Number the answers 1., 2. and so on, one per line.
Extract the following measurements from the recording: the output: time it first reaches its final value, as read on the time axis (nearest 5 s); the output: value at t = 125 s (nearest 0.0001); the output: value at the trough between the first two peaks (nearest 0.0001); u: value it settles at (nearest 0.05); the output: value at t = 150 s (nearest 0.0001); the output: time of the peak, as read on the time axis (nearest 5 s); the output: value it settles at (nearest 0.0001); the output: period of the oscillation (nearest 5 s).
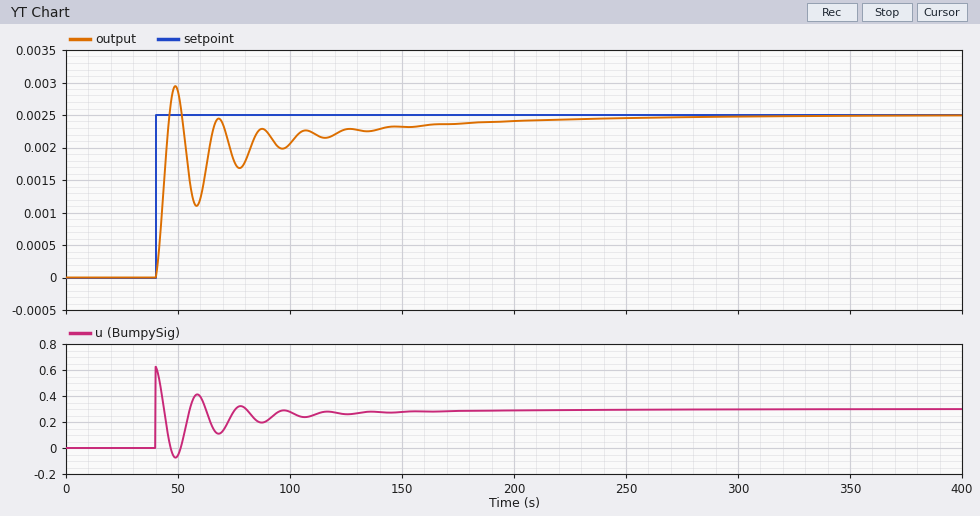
1. 45 s
2. 0.0023
3. 0.0011
4. 0.30
5. 0.0023
6. 50 s
7. 0.0025
8. 20 s
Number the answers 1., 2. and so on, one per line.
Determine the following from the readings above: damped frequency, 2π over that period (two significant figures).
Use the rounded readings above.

1. 0.31 rad/s
